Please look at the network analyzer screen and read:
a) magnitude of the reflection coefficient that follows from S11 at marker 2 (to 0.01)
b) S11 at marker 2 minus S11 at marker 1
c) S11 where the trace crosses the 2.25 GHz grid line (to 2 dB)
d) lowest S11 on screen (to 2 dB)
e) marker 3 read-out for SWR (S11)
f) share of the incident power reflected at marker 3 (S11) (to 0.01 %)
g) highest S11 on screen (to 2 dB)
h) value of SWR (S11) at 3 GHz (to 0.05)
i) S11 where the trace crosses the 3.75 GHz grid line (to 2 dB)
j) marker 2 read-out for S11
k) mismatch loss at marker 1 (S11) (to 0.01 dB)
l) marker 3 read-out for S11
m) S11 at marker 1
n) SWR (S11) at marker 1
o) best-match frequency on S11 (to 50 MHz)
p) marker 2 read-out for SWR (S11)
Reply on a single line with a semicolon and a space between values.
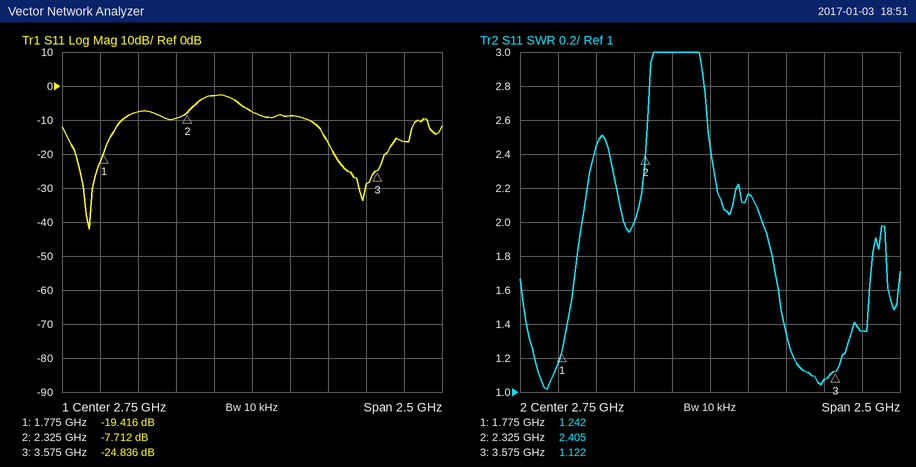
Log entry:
0.41; 11.704 dB; -10 dB; -42 dB; 1.122; 0.33 %; -2 dB; 2.15; -16 dB; -7.712 dB; 0.05 dB; -24.836 dB; -19.416 dB; 1.242; 1.70 GHz; 2.405
